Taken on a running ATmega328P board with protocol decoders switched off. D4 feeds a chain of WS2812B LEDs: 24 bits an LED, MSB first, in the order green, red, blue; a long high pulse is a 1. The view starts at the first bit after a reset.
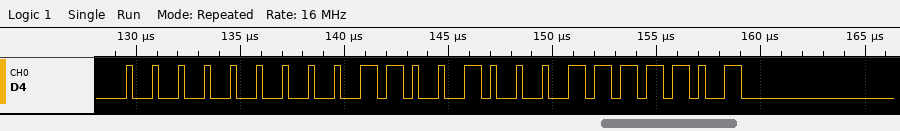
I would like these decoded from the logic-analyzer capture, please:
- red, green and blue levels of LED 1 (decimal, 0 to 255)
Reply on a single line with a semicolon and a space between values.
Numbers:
100, 0, 125
